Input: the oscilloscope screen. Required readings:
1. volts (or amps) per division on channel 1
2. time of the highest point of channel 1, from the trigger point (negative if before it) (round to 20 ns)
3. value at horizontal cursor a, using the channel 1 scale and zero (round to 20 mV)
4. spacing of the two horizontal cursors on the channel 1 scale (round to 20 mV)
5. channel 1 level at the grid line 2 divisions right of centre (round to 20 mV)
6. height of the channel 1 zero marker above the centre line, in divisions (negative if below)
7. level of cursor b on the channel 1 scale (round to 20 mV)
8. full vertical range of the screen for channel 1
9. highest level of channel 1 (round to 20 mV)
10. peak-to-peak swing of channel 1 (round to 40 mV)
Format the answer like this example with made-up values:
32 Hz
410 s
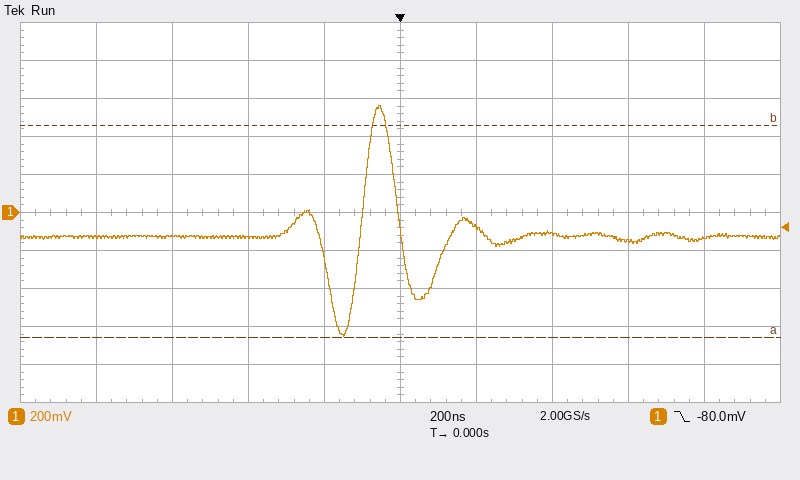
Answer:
200 mV
-60 ns
-660 mV
1.12 V
-120 mV
0.0 div
460 mV
2 V
560 mV
1.20 V
